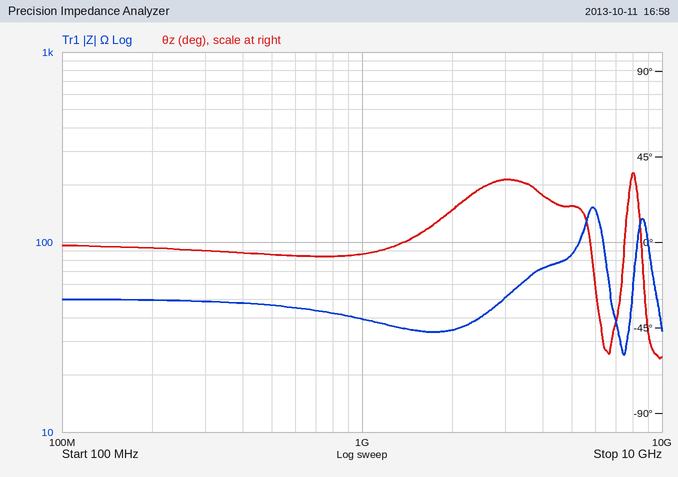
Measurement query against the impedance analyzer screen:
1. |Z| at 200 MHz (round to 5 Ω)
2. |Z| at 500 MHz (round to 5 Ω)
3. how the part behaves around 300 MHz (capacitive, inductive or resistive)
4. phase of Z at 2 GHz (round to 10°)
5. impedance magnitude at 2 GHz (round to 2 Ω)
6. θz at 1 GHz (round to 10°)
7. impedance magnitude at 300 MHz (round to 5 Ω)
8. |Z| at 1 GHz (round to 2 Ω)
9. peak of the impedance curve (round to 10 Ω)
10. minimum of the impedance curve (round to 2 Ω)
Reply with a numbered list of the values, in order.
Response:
1. 50 Ω
2. 45 Ω
3. resistive
4. 20°
5. 34 Ω
6. -10°
7. 50 Ω
8. 40 Ω
9. 150 Ω
10. 26 Ω
